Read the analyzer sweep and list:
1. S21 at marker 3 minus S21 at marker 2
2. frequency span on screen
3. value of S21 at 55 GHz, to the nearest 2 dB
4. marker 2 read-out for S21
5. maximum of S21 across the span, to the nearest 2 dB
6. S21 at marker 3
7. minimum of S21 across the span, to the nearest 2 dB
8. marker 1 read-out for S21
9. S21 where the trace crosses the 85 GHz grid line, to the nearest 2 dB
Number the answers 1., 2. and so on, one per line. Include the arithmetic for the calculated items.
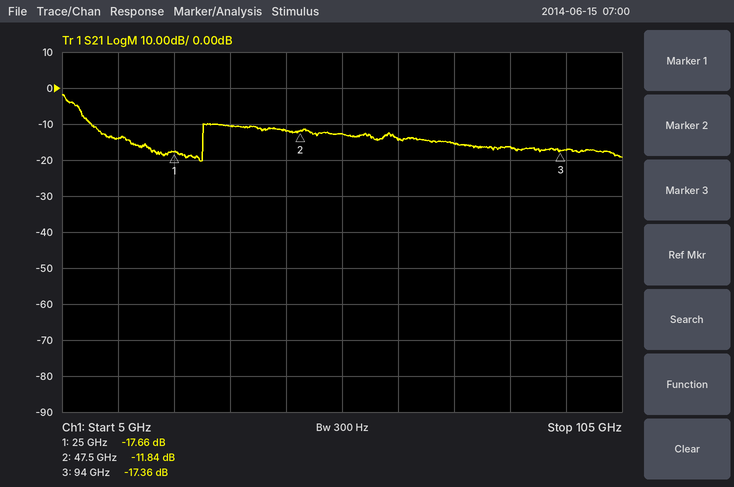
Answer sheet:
1. -17.36 − (-11.84) = -5.52 dB
2. 100 GHz
3. -12 dB
4. -11.84 dB
5. -2 dB
6. -17.36 dB
7. -20 dB
8. -17.66 dB
9. -16 dB
